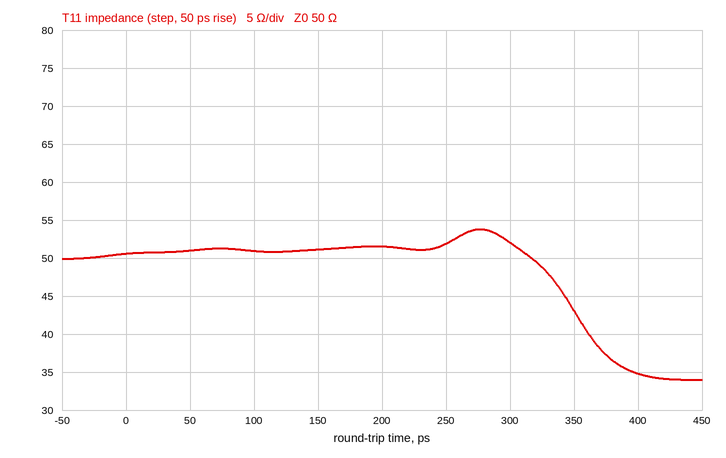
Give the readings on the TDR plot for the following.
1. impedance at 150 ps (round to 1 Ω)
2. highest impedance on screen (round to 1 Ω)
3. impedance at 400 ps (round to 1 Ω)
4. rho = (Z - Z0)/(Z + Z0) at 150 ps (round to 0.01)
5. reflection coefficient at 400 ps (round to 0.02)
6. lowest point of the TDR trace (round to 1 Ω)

51 Ω
54 Ω
35 Ω
+0.01
-0.18
34 Ω
